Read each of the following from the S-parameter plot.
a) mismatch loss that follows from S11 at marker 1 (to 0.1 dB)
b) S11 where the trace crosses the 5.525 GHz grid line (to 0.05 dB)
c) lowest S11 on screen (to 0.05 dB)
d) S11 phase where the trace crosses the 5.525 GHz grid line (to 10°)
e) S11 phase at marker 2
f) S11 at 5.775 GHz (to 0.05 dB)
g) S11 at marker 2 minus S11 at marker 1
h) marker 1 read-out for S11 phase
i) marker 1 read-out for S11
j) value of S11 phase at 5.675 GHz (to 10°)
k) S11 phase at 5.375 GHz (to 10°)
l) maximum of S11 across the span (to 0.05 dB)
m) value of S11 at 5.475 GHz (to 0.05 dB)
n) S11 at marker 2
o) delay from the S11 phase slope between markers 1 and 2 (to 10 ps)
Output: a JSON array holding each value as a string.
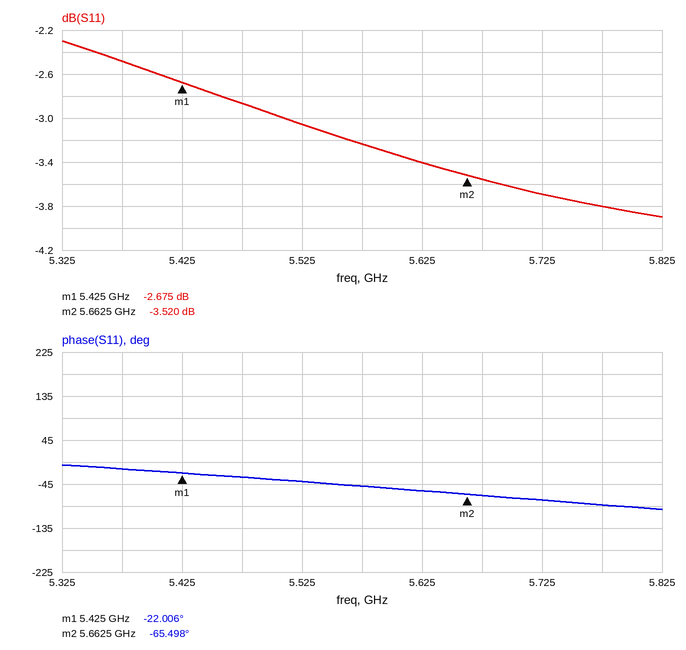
["3.4 dB", "-3.05 dB", "-3.90 dB", "-40°", "-65.498°", "-3.80 dB", "-0.845 dB", "-22.006°", "-2.675 dB", "-70°", "-10°", "-2.30 dB", "-2.85 dB", "-3.520 dB", "510 ps"]
